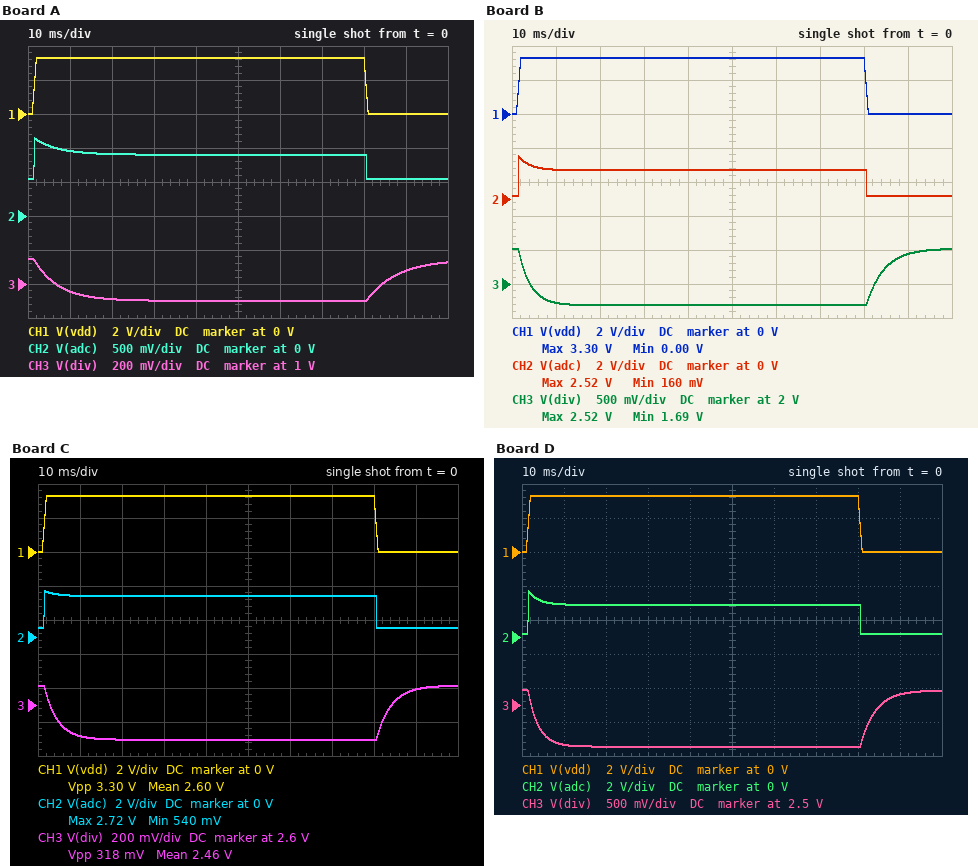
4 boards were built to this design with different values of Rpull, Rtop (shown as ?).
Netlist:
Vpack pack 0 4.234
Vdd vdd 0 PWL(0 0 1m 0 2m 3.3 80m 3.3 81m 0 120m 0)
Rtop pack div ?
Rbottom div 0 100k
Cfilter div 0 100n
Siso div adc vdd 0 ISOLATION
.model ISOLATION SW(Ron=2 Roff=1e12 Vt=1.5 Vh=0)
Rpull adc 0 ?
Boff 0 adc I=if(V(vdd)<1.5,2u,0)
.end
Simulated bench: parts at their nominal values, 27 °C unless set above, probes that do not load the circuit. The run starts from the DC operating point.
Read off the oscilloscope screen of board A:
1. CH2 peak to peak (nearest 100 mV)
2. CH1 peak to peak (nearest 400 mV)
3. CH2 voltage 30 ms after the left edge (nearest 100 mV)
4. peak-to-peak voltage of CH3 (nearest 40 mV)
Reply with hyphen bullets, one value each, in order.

- 600 mV
- 3.2 V
- 900 mV
- 240 mV
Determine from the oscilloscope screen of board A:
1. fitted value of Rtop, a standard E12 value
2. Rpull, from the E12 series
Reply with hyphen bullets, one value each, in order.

- 270 kΩ
- 270 kΩ
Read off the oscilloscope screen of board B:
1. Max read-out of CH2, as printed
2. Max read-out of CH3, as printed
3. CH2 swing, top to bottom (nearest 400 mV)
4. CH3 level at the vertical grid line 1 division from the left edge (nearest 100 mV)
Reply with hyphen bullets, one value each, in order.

- 2.52 V
- 2.52 V
- 2.4 V
- 1.7 V
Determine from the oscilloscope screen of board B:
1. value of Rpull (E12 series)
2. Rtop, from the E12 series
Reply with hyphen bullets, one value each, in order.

- 82 kΩ
- 68 kΩ
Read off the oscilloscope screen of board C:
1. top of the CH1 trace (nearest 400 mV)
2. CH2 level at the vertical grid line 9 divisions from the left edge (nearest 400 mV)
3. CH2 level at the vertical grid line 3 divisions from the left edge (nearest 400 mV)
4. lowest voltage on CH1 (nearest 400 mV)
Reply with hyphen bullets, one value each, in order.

- 3.2 V
- 400 mV
- 2.4 V
- 0 V
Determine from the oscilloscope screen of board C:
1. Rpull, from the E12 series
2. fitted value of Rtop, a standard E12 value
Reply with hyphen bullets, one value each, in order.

- 270 kΩ
- 56 kΩ
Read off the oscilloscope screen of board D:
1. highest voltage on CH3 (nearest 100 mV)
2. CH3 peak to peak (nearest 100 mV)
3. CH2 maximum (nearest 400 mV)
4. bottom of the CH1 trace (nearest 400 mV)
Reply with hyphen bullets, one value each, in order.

- 2.7 V
- 800 mV
- 2.8 V
- 0 V
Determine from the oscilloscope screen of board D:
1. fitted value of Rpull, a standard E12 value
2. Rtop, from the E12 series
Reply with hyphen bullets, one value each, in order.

- 82 kΩ
- 56 kΩ
